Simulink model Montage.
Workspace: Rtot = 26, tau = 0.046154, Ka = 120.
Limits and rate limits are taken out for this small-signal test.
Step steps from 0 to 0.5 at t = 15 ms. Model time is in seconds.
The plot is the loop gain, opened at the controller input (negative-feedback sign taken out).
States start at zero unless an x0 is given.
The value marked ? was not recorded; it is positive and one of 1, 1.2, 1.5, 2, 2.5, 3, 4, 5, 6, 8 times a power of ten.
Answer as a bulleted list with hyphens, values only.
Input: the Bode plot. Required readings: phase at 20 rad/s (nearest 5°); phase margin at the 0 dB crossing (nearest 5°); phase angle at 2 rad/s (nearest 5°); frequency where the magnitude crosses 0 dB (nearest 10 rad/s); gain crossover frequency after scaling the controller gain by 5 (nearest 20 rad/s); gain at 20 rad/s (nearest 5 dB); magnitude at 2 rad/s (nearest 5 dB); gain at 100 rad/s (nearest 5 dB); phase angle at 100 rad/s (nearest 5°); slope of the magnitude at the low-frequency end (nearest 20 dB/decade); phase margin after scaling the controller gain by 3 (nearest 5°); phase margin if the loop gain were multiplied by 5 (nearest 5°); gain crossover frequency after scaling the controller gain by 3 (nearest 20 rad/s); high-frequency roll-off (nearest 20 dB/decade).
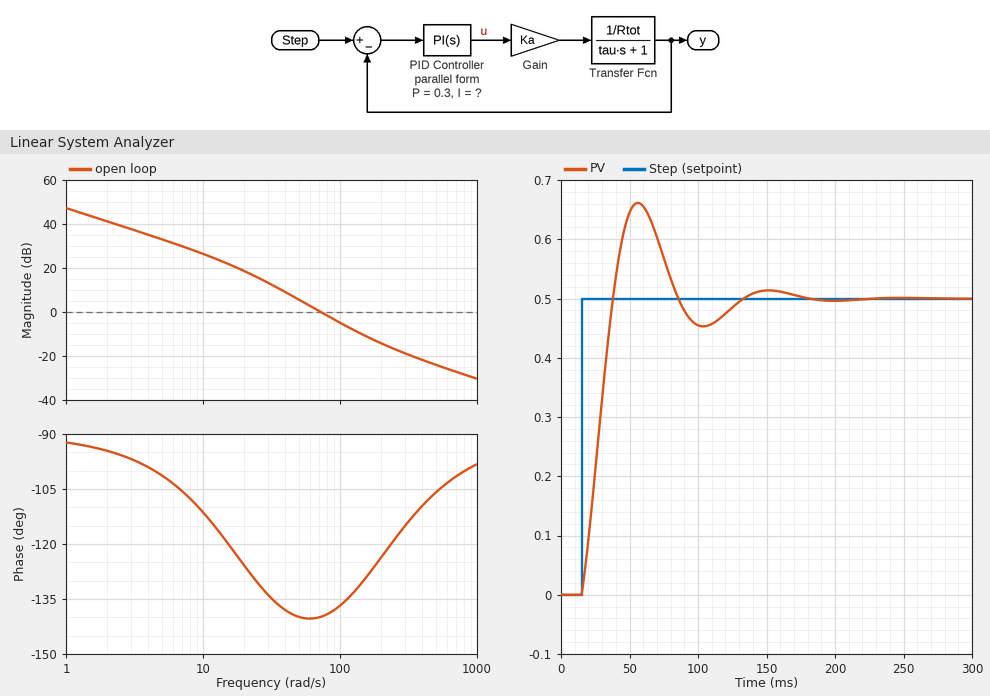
- -125°
- 40°
- -95°
- 70 rad/s
- 200 rad/s
- 20 dB
- 40 dB
- -5 dB
- -135°
- -20 dB/decade
- 50°
- 55°
- 140 rad/s
- -20 dB/decade
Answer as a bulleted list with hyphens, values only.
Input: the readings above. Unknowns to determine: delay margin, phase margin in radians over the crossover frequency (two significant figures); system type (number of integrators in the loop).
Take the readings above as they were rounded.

- 0.0100 s
- 1
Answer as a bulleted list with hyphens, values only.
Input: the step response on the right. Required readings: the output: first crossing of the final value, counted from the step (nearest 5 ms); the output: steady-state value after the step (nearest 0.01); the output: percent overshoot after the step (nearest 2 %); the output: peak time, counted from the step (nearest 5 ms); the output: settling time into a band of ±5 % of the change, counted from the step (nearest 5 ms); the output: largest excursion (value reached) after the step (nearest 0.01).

- 25 ms
- 0.50
- 32 %
- 40 ms
- 105 ms
- 0.66
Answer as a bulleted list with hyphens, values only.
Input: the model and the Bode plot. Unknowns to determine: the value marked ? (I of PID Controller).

- 50
